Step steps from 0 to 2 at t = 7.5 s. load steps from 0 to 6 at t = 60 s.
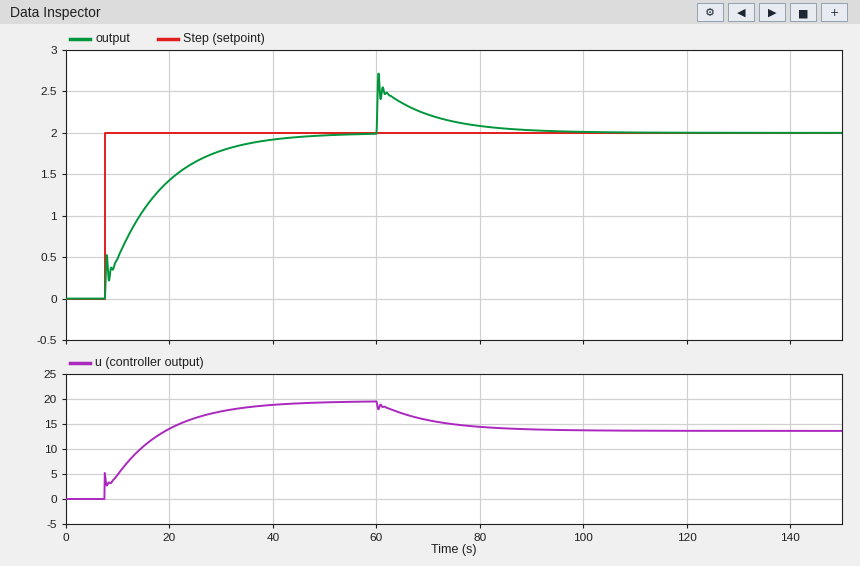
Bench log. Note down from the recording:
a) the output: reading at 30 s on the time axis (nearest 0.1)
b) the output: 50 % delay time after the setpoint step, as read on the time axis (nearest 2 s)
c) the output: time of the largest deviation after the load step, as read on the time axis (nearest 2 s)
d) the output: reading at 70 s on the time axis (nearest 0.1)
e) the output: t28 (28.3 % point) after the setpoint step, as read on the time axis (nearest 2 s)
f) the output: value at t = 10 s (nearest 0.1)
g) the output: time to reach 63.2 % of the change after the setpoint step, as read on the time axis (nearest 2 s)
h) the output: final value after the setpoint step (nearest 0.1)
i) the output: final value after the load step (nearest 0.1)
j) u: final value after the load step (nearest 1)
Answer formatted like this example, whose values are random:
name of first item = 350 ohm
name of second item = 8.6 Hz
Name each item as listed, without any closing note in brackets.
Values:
the output: reading at 30 s on the time axis = 1.8
the output: 50 % delay time after the setpoint step, as read on the time axis = 14 s
the output: time of the largest deviation after the load step, as read on the time axis = 60 s
the output: reading at 70 s on the time axis = 2.2
the output: t28 (28.3 % point) after the setpoint step, as read on the time axis = 10 s
the output: value at t = 10 s = 0.5
the output: time to reach 63.2 % of the change after the setpoint step, as read on the time axis = 18 s
the output: final value after the setpoint step = 2.0
the output: final value after the load step = 2.0
u: final value after the load step = 14
